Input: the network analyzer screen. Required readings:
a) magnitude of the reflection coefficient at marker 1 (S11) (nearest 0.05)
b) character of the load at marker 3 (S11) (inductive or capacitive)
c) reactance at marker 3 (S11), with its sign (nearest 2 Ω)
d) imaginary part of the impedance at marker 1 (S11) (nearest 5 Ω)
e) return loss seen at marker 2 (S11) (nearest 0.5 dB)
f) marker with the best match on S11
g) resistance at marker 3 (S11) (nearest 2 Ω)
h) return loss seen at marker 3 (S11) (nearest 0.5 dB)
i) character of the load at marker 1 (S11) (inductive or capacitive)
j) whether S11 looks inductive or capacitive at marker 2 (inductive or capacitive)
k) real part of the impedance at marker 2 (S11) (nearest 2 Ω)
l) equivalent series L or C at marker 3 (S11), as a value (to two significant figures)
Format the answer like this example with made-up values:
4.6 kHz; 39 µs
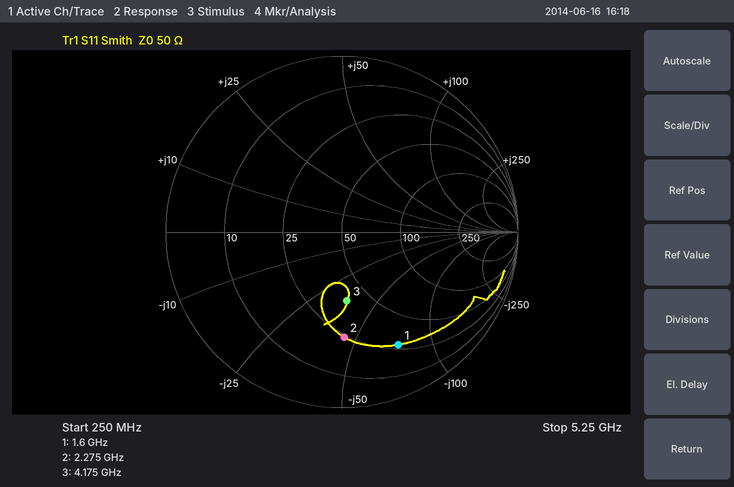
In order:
0.70; capacitive; -36 Ω; -75 Ω; 4.5 dB; marker 3; 38 Ω; 8.0 dB; capacitive; capacitive; 24 Ω; 1.1 pF
